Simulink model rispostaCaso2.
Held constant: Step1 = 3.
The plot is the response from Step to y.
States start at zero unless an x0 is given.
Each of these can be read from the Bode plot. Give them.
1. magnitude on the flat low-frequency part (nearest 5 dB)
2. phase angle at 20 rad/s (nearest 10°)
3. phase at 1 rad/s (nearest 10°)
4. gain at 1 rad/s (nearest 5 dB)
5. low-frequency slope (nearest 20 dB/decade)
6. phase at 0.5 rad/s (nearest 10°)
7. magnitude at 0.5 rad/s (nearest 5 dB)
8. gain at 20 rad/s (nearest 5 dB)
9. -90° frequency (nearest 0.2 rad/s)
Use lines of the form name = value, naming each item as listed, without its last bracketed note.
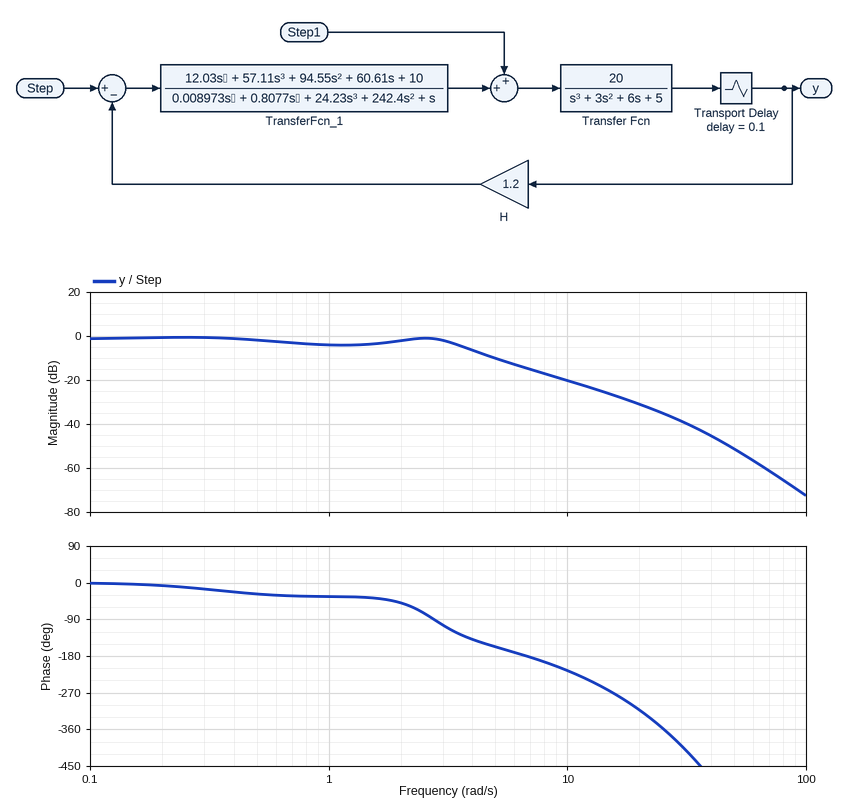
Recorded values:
magnitude on the flat low-frequency part = 0 dB
phase angle at 20 rad/s = -310°
phase at 1 rad/s = -30°
gain at 1 rad/s = -5 dB
low-frequency slope = 0 dB/decade
phase at 0.5 rad/s = -30°
magnitude at 0.5 rad/s = 0 dB
gain at 20 rad/s = -30 dB
-90° frequency = 2.8 rad/s
